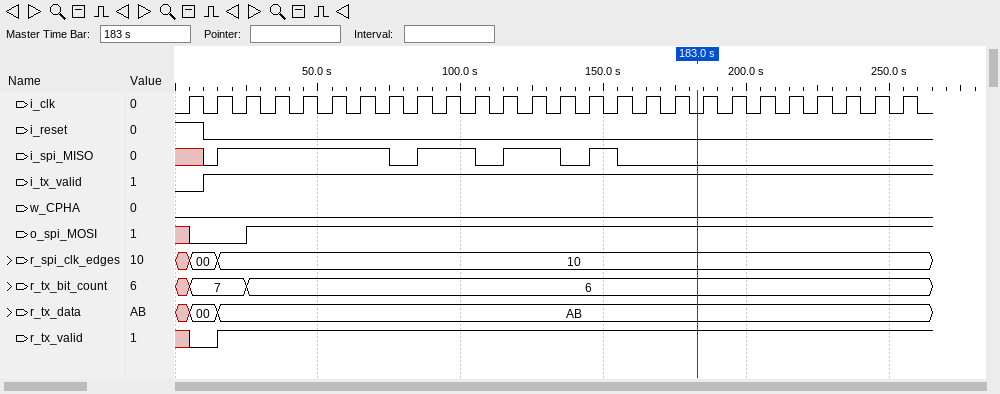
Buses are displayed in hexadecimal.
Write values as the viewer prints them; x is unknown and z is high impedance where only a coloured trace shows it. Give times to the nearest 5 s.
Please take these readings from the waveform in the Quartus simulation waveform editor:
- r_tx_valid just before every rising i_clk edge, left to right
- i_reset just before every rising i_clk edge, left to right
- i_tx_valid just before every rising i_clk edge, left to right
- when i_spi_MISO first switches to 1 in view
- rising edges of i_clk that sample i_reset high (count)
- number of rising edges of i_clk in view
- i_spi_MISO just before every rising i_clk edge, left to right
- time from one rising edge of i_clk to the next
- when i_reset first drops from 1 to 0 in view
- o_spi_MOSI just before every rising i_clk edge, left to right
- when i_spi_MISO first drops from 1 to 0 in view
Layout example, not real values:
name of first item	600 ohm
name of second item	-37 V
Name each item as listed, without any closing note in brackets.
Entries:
r_tx_valid just before every rising i_clk edge, left to right	x 0 1 1 1 1 1 1 1 1 1 1 1 1 1 1 1 1 1 1 1 1 1 1 1 1
i_reset just before every rising i_clk edge, left to right	1 0 0 0 0 0 0 0 0 0 0 0 0 0 0 0 0 0 0 0 0 0 0 0 0 0
i_tx_valid just before every rising i_clk edge, left to right	0 1 1 1 1 1 1 1 1 1 1 1 1 1 1 1 1 1 1 1 1 1 1 1 1 1
when i_spi_MISO first switches to 1 in view	15 s
rising edges of i_clk that sample i_reset high	1
number of rising edges of i_clk in view	26
i_spi_MISO just before every rising i_clk edge, left to right	x 0 1 1 1 1 1 1 0 1 1 0 1 1 0 1 0 0 0 0 0 0 0 0 0 0
time from one rising edge of i_clk to the next	10 s
when i_reset first drops from 1 to 0 in view	10 s
o_spi_MOSI just before every rising i_clk edge, left to right	x 0 0 1 1 1 1 1 1 1 1 1 1 1 1 1 1 1 1 1 1 1 1 1 1 1
when i_spi_MISO first drops from 1 to 0 in view	75 s
